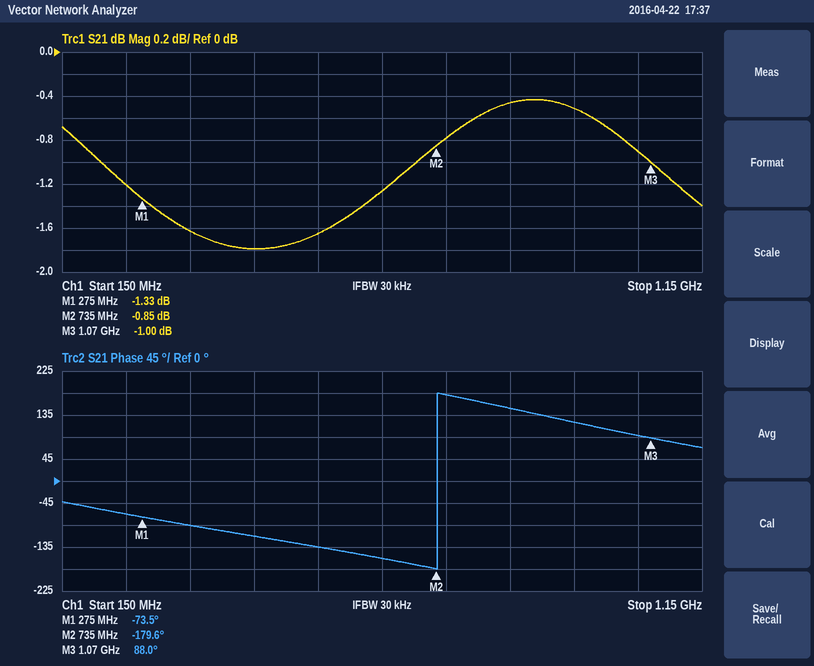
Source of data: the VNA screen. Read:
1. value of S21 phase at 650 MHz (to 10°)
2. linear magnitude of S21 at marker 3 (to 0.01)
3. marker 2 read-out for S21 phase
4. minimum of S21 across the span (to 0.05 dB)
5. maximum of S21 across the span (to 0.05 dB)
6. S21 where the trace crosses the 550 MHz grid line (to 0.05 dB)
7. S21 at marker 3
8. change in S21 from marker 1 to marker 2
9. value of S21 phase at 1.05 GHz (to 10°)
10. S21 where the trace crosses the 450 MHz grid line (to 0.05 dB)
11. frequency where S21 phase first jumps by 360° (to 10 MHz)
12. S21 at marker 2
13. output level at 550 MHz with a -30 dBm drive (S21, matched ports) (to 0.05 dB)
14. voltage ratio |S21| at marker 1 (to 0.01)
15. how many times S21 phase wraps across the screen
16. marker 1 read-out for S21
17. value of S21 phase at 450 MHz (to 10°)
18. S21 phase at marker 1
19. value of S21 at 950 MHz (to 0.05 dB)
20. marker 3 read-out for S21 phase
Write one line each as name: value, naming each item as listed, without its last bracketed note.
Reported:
value of S21 phase at 650 MHz: -160°
linear magnitude of S21 at marker 3: 0.89
marker 2 read-out for S21 phase: -179.6°
minimum of S21 across the span: -1.80 dB
maximum of S21 across the span: -0.45 dB
S21 where the trace crosses the 550 MHz grid line: -1.65 dB
S21 at marker 3: -1.00 dB
change in S21 from marker 1 to marker 2: 0.48 dB
value of S21 phase at 1.05 GHz: 90°
S21 where the trace crosses the 450 MHz grid line: -1.80 dB
frequency where S21 phase first jumps by 360°: 740 MHz
S21 at marker 2: -0.85 dB
output level at 550 MHz with a -30 dBm drive (S21, matched ports): -31.65 dBm
voltage ratio |S21| at marker 1: 0.86
how many times S21 phase wraps across the screen: 1
marker 1 read-out for S21: -1.33 dB
value of S21 phase at 450 MHz: -110°
S21 phase at marker 1: -73.5°
value of S21 at 950 MHz: -0.50 dB
marker 3 read-out for S21 phase: 88.0°
